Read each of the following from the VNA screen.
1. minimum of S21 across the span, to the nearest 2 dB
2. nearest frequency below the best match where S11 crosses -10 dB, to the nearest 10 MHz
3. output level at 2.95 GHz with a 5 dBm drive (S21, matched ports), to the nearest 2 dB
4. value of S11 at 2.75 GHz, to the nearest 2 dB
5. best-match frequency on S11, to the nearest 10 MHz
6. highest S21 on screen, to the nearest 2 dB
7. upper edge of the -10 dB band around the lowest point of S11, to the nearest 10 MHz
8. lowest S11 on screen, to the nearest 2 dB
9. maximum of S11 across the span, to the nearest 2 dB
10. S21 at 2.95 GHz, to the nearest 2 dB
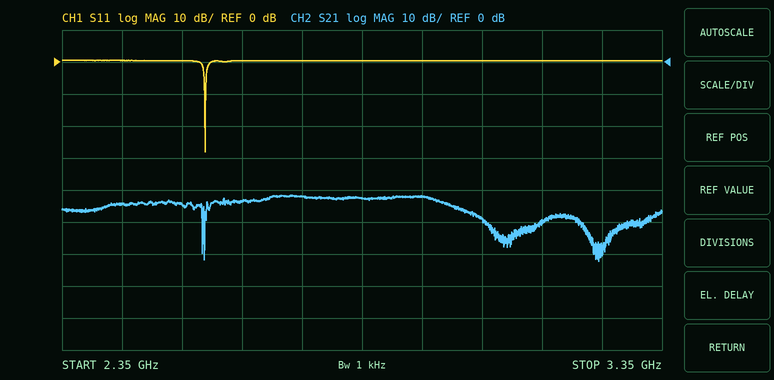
-62 dB
2.59 GHz
-38 dBm
0 dB
2.59 GHz
-42 dB
2.59 GHz
-28 dB
0 dB
-42 dB
